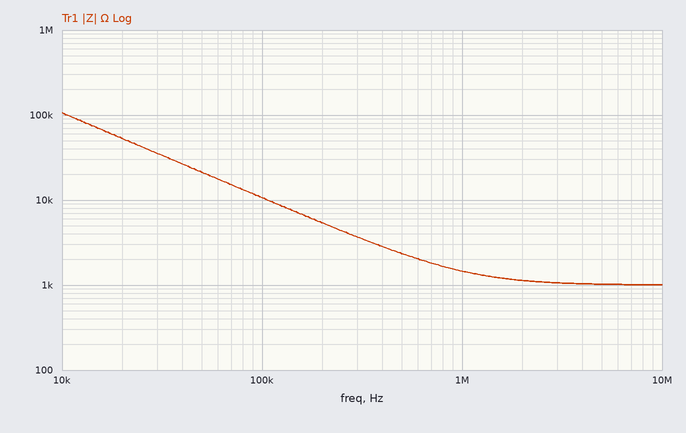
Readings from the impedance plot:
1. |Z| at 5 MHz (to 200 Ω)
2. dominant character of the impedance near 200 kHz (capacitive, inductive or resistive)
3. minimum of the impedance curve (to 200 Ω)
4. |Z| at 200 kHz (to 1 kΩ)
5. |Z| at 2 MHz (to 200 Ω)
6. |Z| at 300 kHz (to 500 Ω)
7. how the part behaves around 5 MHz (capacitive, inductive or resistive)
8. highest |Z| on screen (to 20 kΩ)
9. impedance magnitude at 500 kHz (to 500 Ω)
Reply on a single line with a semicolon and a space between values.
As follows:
1.0 kΩ; capacitive; 1.0 kΩ; 5 kΩ; 1.2 kΩ; 3.5 kΩ; resistive; 100 kΩ; 2.5 kΩ
